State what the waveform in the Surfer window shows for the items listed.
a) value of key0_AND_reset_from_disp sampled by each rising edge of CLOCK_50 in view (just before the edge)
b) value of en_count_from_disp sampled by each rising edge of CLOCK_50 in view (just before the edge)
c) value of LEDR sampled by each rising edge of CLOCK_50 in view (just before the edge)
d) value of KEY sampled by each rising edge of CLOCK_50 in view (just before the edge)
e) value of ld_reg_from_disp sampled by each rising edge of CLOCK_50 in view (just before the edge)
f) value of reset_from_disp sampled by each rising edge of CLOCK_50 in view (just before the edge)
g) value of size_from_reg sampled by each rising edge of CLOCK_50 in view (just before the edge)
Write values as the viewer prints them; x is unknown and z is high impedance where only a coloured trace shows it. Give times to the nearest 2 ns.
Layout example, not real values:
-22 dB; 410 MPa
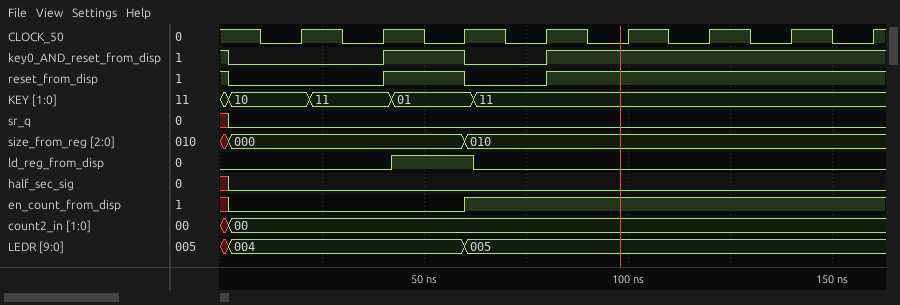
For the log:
0 0 1 0 1 1 1 1; 0 0 0 1 1 1 1 1; 004, 004, 004, 005, 005, 005, 005, 005; 10, 11, 01, 11, 11, 11, 11, 11; 0 0 1 0 0 0 0 0; 0 0 1 0 1 1 1 1; 000, 000, 000, 010, 010, 010, 010, 010
